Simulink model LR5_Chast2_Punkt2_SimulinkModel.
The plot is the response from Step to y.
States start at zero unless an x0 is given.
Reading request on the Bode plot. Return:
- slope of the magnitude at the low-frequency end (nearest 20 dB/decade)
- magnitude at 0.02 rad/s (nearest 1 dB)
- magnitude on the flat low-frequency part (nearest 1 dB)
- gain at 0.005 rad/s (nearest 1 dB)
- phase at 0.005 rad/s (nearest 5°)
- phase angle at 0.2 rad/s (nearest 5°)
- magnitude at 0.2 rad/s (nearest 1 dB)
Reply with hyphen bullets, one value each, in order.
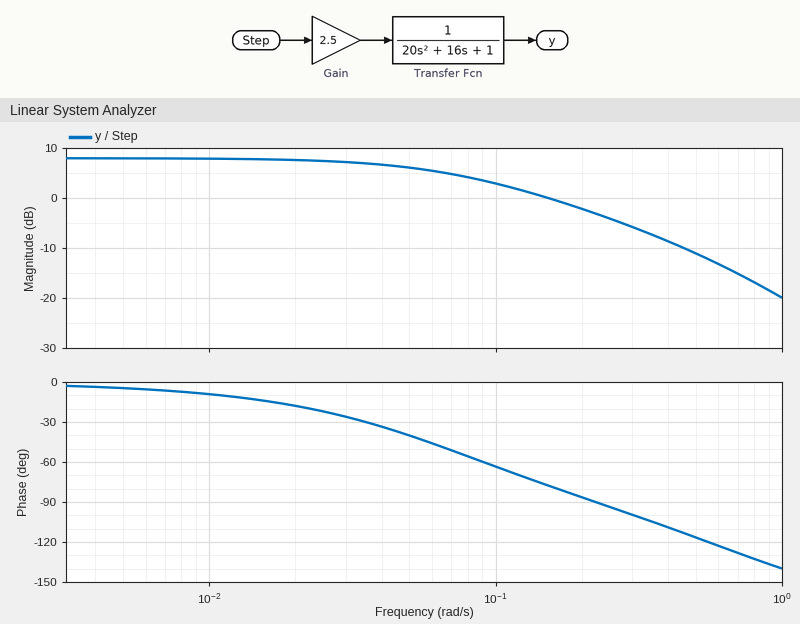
- 0 dB/decade
- 8 dB
- 8 dB
- 8 dB
- -5°
- -85°
- -2 dB
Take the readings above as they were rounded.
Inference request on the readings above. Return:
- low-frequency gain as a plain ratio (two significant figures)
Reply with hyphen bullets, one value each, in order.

- 2.5
